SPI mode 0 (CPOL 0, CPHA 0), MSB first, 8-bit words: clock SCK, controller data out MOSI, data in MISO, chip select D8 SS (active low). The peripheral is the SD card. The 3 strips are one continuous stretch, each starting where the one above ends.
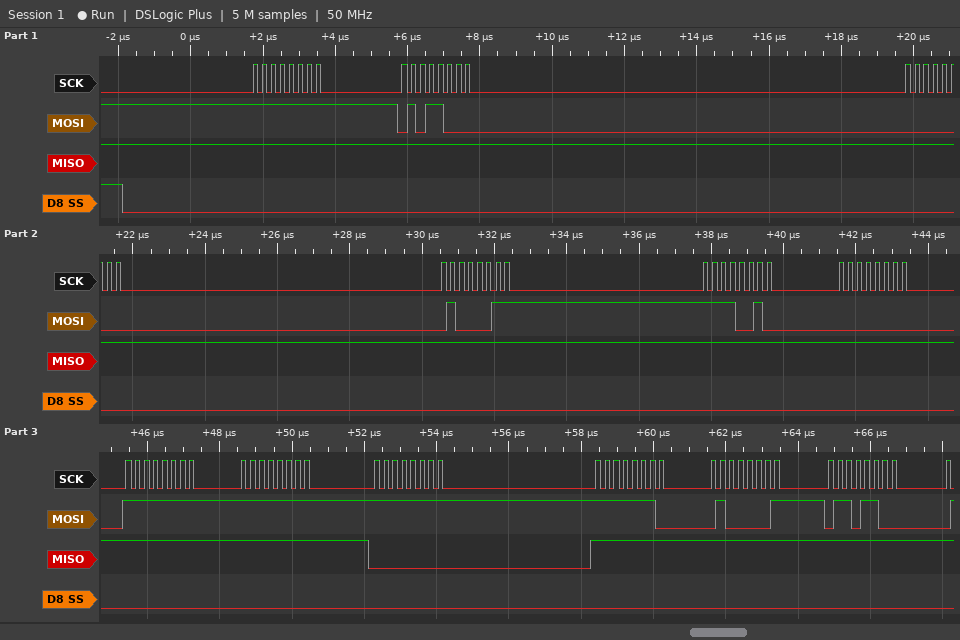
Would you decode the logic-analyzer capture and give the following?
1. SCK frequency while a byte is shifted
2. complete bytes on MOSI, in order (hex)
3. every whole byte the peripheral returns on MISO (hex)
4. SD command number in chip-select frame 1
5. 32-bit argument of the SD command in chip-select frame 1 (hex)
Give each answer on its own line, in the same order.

4 MHz
FF 58 00 43 F2 00 FF FF FF FE 41 6C
FF FF FF FF FF FF FF FF 00 FF FF FF
CMD24
0x0043F200
